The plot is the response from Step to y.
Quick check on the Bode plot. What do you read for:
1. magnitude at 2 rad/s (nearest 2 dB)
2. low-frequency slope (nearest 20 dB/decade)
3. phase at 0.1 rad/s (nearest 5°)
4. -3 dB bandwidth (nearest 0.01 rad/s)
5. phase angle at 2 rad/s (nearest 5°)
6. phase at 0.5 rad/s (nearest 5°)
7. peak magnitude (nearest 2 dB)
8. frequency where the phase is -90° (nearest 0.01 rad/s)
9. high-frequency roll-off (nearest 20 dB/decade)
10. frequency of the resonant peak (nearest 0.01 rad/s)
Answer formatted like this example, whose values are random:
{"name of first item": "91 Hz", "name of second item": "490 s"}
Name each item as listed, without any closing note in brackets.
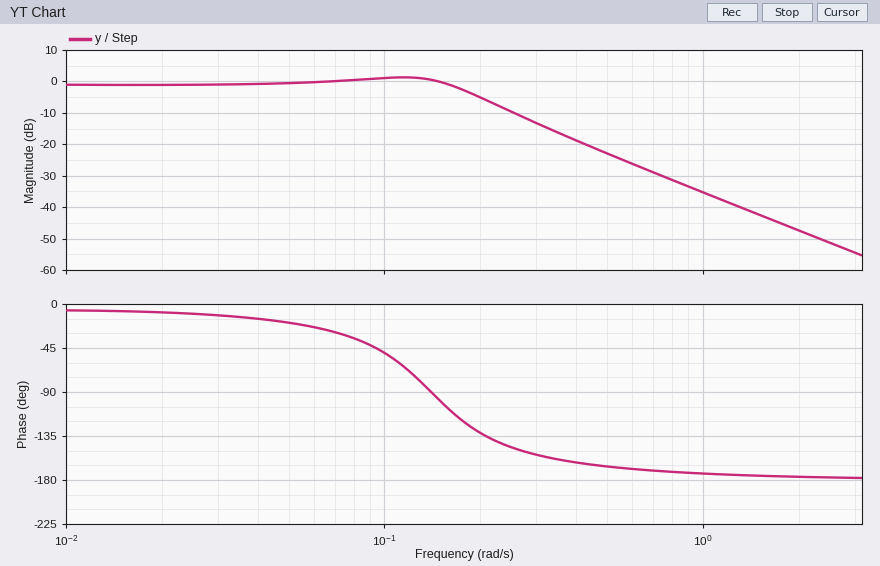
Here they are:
{"magnitude at 2 rad/s": "-48 dB", "low-frequency slope": "0 dB/decade", "phase at 0.1 rad/s": "-50°", "-3 dB bandwidth": "0.19 rad/s", "phase angle at 2 rad/s": "-175°", "phase at 0.5 rad/s": "-165°", "peak magnitude": "2 dB", "frequency where the phase is -90°": "0.14 rad/s", "high-frequency roll-off": "-40 dB/decade", "frequency of the resonant peak": "0.11 rad/s"}
